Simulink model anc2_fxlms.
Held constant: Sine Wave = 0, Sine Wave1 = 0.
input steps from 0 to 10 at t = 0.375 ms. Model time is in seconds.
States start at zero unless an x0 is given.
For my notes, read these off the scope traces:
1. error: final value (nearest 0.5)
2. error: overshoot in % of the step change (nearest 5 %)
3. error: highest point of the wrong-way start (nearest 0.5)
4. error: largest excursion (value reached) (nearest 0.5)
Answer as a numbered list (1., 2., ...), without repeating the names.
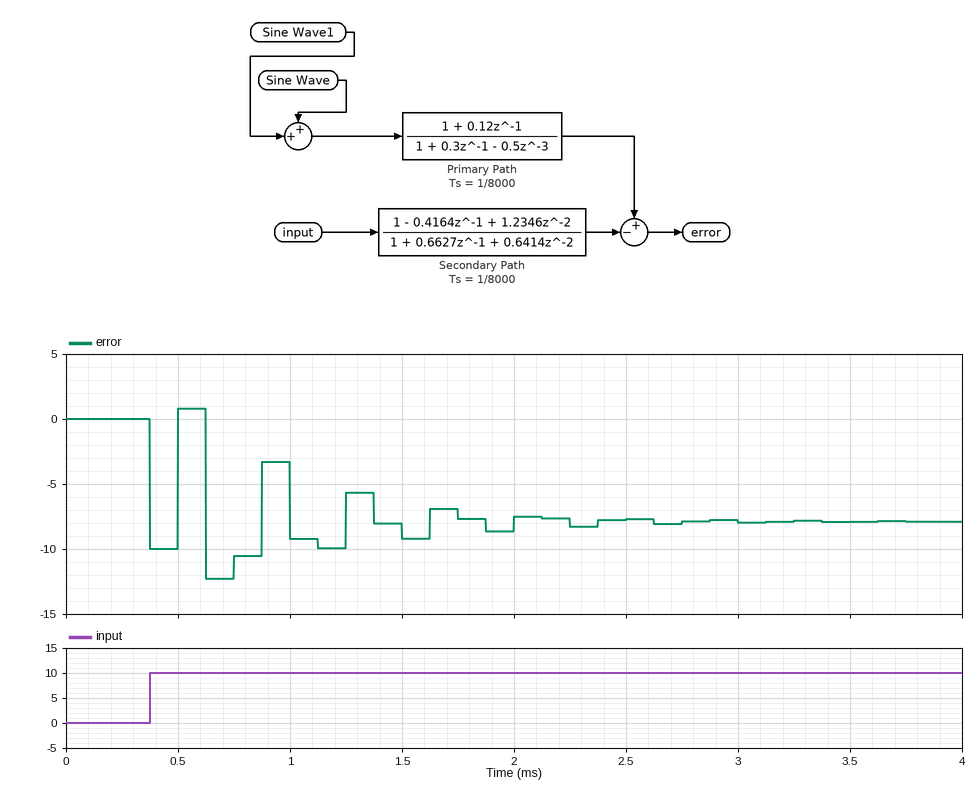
1. -8.0
2. 55 %
3. 1.0
4. -12.5
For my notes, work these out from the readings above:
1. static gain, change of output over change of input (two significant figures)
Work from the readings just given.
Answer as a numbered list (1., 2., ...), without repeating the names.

1. -0.80
